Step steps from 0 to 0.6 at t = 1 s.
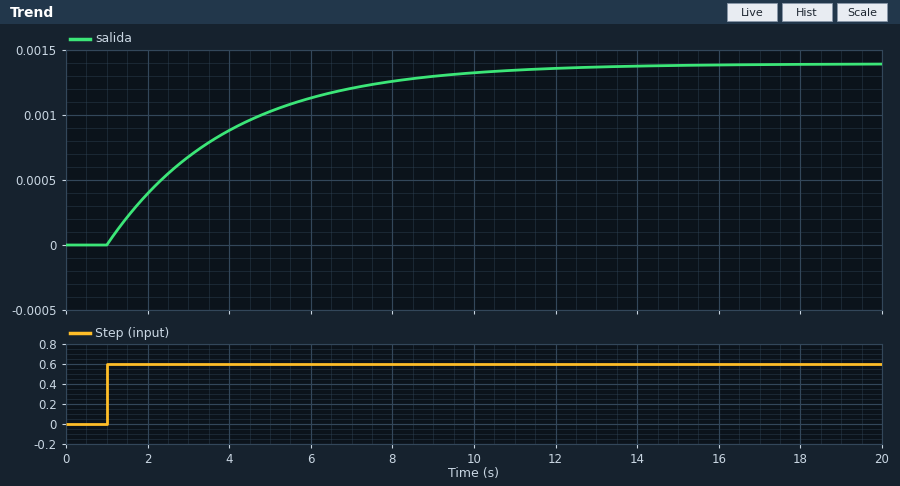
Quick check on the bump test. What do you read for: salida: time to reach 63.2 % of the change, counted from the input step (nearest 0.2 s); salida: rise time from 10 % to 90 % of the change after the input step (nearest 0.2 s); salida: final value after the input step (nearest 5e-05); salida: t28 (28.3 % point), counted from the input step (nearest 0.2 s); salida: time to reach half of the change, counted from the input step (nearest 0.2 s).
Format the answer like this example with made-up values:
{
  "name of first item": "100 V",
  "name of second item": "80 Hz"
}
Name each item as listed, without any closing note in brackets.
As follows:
{
  "salida: time to reach 63.2 % of the change, counted from the input step": "3.0 s",
  "salida: rise time from 10 % to 90 % of the change after the input step": "6.6 s",
  "salida: final value after the input step": "0.00140",
  "salida: t28 (28.3 % point), counted from the input step": "1.0 s",
  "salida: time to reach half of the change, counted from the input step": "2.0 s"
}
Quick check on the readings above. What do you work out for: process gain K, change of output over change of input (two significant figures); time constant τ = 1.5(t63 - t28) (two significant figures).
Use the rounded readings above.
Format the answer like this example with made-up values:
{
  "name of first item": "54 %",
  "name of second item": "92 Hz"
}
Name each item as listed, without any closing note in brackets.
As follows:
{
  "process gain K, change of output over change of input": "0.0023",
  "time constant τ = 1.5(t63 - t28)": "3.0 s"
}
